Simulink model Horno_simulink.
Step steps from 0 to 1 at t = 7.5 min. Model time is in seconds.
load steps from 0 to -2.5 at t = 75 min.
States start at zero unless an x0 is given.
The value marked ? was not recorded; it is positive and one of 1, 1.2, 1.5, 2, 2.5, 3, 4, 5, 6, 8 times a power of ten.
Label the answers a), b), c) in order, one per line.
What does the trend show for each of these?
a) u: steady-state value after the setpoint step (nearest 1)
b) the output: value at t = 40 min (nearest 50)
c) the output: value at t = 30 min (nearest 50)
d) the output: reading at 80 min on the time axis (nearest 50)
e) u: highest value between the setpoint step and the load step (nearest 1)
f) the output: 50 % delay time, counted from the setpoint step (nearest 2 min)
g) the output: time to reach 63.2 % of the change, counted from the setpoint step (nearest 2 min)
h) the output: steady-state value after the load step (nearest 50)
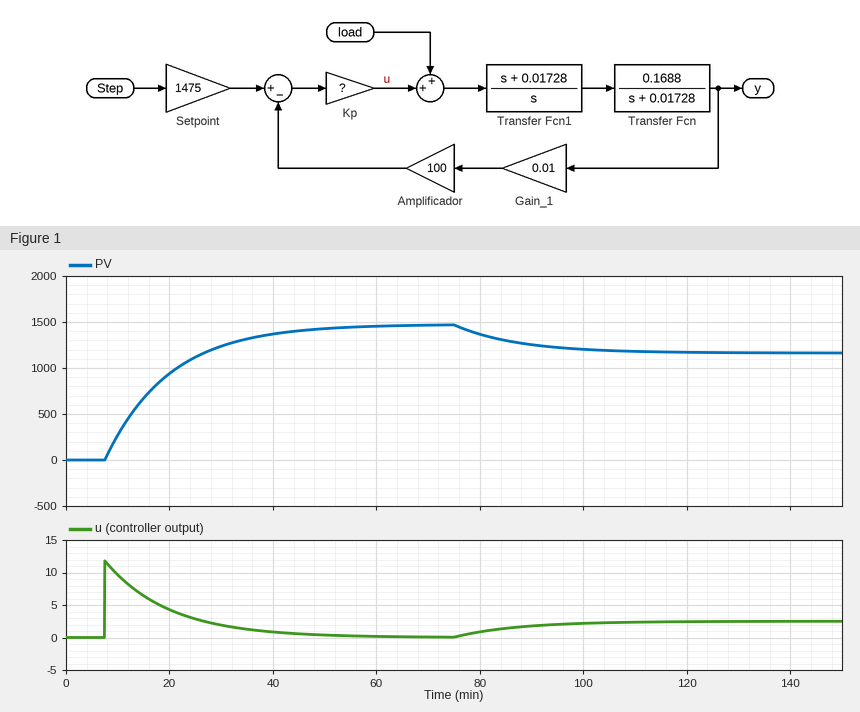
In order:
a) 0
b) 1350
c) 1250
d) 1350
e) 12
f) 8 min
g) 12 min
h) 1150
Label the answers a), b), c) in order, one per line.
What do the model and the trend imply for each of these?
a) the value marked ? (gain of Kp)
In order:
a) 0.008
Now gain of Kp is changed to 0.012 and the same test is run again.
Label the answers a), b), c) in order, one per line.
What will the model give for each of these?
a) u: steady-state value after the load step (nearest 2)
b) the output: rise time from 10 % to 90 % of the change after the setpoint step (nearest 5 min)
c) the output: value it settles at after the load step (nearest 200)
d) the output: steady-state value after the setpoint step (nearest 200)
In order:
a) 2
b) 20 min
c) 1200
d) 1400
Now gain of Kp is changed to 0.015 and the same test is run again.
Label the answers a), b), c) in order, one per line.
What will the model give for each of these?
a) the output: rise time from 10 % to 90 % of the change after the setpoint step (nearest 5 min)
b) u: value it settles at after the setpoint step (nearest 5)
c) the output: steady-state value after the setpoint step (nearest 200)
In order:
a) 15 min
b) 0
c) 1400
